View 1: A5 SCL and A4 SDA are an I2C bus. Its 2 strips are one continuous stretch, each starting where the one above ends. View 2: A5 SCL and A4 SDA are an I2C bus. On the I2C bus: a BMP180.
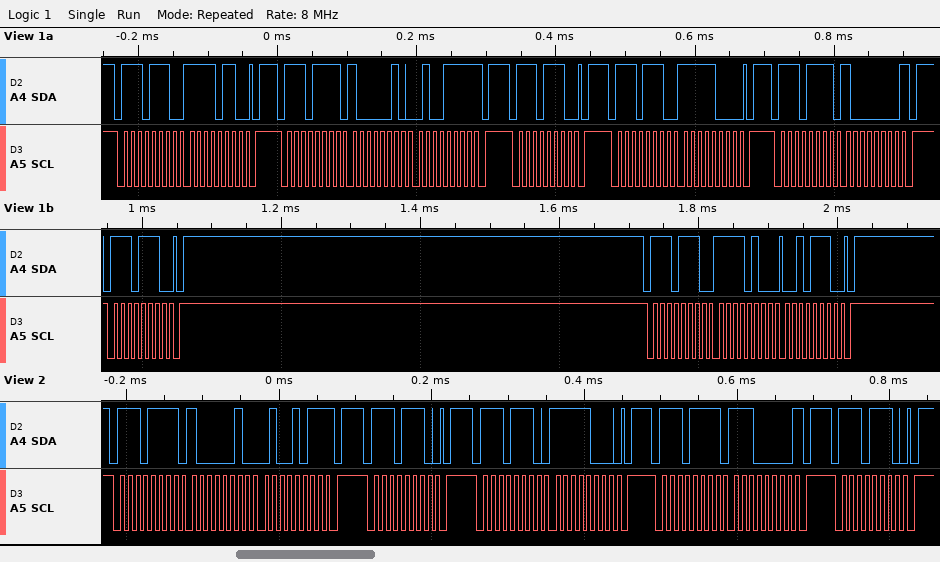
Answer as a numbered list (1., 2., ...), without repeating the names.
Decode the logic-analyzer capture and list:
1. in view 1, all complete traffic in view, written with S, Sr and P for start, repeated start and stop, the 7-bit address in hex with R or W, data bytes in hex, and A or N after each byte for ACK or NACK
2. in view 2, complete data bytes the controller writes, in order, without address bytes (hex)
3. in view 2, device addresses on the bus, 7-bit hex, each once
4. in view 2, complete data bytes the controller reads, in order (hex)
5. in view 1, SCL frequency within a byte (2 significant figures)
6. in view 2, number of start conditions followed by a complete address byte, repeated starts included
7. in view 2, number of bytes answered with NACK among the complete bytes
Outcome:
1. S 77W A F6 A P S 77R A 82 A 4F N P S 77W A P S 77W A F8 A P S 77R A 80 N P S 77W A P S 77W A F4 A 2E A P
2. F8
3. 0x77
4. 82 4B E0
5. 100 kHz
6. 5
7. 2
